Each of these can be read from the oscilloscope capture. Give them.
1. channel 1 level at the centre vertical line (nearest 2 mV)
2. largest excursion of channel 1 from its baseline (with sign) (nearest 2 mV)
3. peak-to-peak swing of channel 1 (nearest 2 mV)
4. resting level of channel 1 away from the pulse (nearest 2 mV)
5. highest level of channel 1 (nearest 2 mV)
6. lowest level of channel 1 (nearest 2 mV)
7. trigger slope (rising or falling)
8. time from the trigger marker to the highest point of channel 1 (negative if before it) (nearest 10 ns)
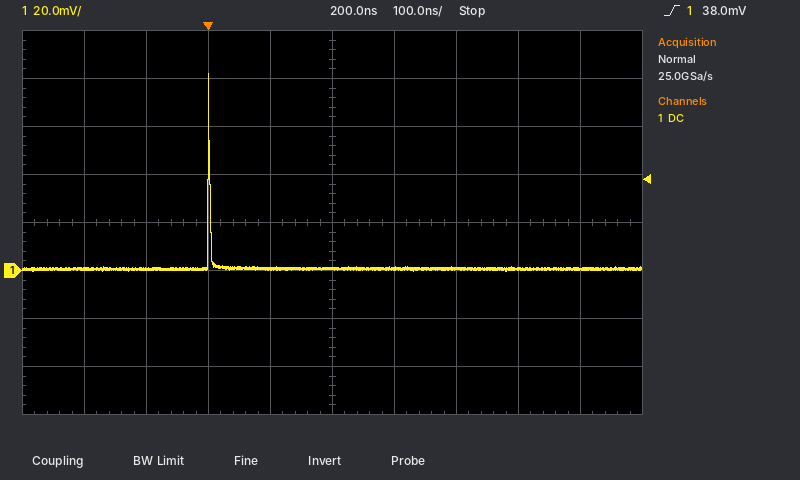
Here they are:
0 mV
+82 mV
82 mV
0 mV
82 mV
0 mV
rising
0 ns
